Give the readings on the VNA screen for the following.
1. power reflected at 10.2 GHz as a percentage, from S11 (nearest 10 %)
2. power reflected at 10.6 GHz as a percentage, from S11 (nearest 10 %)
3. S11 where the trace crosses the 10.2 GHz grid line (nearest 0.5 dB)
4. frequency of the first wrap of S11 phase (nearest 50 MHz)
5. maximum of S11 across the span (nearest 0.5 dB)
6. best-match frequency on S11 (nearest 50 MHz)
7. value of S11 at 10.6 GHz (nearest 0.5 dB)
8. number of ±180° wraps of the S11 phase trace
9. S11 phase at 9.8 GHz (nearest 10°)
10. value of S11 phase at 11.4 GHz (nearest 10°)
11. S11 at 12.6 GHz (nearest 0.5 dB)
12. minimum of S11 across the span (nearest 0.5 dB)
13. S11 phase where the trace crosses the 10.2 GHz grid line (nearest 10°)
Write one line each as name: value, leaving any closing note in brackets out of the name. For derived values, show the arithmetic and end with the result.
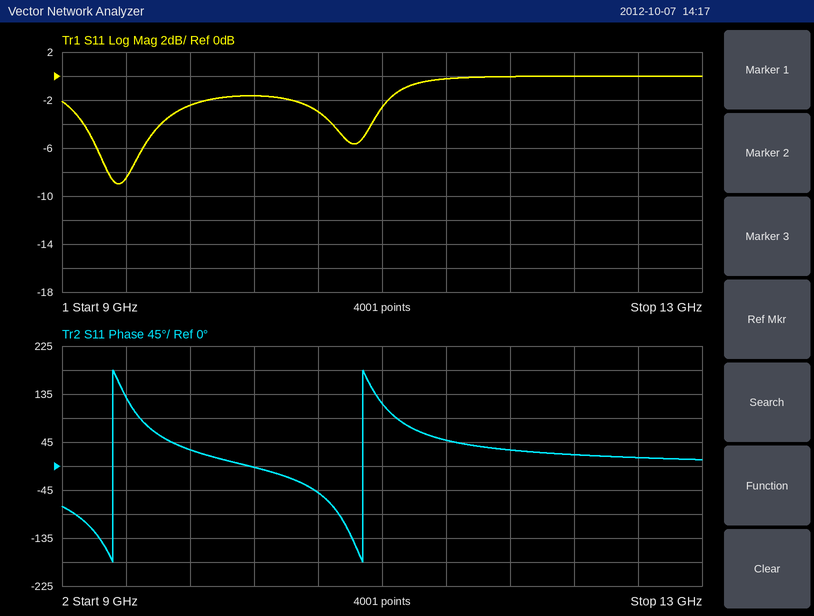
power reflected at 10.2 GHz as a percentage, from S11: 10^(-1.5/10) ≈ 70.8 %, so 70 % to the nearest 10 %
power reflected at 10.6 GHz as a percentage, from S11: 10^(-3/10) ≈ 50 %
S11 where the trace crosses the 10.2 GHz grid line: -1.5 dB
frequency of the first wrap of S11 phase: 9.30 GHz
maximum of S11 across the span: 0.0 dB
best-match frequency on S11: 9.35 GHz
value of S11 at 10.6 GHz: -3.0 dB
number of ±180° wraps of the S11 phase trace: 2
S11 phase at 9.8 GHz: 30°
value of S11 phase at 11.4 GHz: 50°
S11 at 12.6 GHz: 0.0 dB
minimum of S11 across the span: -9.0 dB
S11 phase where the trace crosses the 10.2 GHz grid line: 0°
